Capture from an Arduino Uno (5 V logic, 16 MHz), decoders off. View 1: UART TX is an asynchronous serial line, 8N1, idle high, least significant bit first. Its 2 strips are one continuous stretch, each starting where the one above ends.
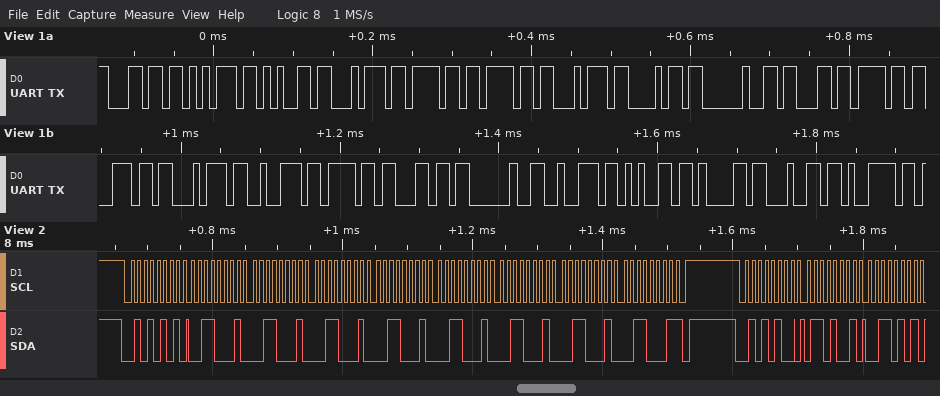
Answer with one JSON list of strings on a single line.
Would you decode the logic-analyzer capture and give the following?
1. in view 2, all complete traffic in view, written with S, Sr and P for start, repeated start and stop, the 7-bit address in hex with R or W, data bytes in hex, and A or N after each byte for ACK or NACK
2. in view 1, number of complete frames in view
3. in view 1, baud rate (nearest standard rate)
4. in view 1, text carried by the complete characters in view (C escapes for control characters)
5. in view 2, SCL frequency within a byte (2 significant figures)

["S 2AR A 31 A 31 A 31 A 31 A 31 A 31 A 31 A 31 N P S 2AW A 69 A 35 A", "22", "115200 baud", "\"luetooth control ready\"", "100 kHz"]
